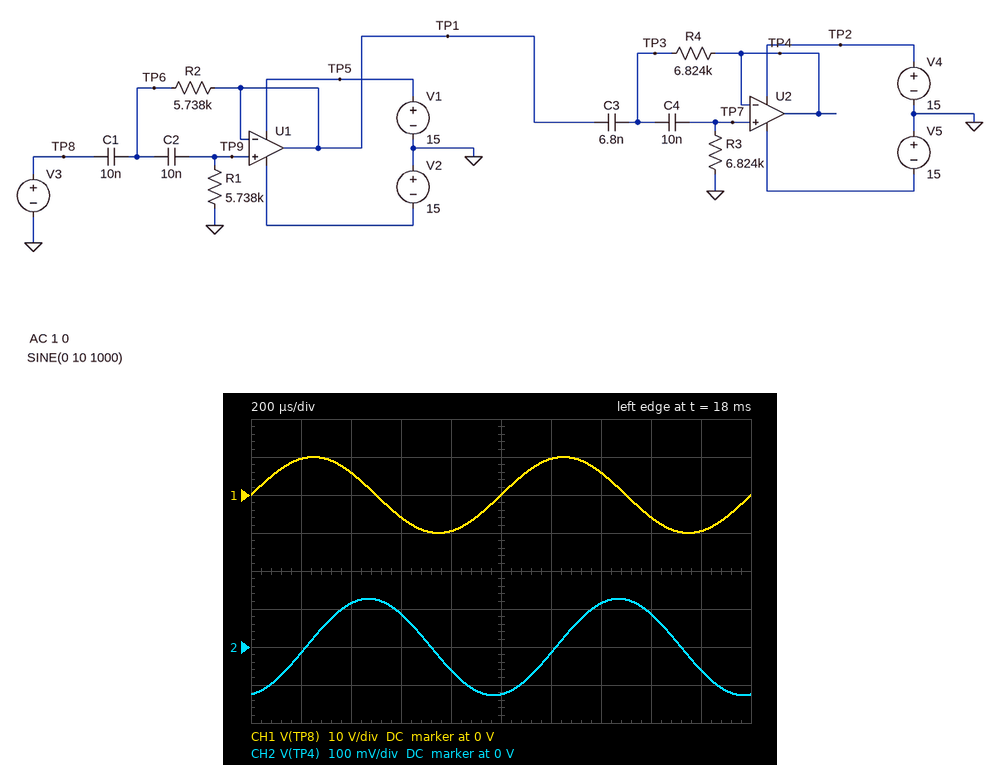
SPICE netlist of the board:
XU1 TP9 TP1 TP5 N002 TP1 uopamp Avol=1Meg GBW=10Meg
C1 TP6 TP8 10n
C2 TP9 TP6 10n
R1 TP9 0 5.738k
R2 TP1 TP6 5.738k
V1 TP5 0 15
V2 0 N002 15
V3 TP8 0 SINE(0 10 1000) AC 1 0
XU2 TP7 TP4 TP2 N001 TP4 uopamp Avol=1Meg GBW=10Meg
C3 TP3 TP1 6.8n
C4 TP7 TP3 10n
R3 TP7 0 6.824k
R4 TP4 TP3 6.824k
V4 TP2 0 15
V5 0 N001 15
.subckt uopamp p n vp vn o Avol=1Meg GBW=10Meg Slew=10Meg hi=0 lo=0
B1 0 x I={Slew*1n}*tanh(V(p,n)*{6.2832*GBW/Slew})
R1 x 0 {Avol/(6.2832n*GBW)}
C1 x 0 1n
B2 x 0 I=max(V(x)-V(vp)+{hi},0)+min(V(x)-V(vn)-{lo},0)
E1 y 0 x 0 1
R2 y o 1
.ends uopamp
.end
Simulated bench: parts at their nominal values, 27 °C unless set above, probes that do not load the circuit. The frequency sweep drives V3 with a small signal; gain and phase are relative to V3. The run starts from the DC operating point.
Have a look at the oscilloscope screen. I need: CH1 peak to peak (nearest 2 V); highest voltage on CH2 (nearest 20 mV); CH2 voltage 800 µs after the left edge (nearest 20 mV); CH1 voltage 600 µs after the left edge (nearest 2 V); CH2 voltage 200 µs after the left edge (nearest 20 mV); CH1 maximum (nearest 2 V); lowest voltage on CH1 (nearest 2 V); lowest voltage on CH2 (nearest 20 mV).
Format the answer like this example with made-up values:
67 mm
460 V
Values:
20 V
120 mV
-60 mV
-6 V
-20 mV
10 V
-10 V
-120 mV
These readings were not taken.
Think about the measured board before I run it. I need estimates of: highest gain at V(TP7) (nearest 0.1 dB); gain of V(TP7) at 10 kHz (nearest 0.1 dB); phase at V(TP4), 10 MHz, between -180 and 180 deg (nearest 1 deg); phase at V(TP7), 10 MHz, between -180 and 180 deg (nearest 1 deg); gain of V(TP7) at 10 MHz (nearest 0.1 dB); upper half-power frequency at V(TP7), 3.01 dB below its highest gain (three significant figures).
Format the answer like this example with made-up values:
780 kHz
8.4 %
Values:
0 dB
-1.4 dB
-90 deg
-45 deg
-3.0 dB
10.0 MHz
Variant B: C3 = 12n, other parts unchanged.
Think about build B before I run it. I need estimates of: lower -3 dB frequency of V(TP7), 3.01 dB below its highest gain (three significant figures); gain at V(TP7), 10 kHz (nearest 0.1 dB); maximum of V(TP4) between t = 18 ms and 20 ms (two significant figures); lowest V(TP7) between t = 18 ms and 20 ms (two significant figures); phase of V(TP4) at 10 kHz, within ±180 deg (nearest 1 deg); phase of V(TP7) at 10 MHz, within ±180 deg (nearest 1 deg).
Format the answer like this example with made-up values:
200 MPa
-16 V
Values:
5.68 kHz
-1.0 dB
210 mV
-210 mV
55 deg
-45 deg
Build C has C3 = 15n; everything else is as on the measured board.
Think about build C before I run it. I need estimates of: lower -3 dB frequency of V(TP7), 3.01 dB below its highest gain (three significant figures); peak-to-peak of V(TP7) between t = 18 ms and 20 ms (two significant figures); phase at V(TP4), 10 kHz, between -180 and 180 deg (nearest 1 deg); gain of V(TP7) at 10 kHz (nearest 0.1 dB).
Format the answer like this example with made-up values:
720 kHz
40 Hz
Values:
5.50 kHz
490 mV
53 deg
-1.0 dB
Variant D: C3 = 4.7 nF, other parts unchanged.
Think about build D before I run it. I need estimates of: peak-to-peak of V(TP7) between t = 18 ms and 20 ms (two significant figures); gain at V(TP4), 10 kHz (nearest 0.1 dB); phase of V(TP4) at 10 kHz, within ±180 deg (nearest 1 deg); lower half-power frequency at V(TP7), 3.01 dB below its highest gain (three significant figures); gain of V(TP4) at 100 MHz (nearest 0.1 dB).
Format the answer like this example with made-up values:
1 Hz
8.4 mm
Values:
180 mV
-1.8 dB
70 deg
7.60 kHz
-40.1 dB
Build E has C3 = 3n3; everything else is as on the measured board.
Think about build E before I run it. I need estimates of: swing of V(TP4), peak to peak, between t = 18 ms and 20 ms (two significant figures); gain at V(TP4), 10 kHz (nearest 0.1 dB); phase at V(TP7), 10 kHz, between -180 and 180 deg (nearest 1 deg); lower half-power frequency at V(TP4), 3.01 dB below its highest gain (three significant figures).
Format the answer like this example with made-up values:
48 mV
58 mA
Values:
130 mV
-2.6 dB
79 deg
9.23 kHz
